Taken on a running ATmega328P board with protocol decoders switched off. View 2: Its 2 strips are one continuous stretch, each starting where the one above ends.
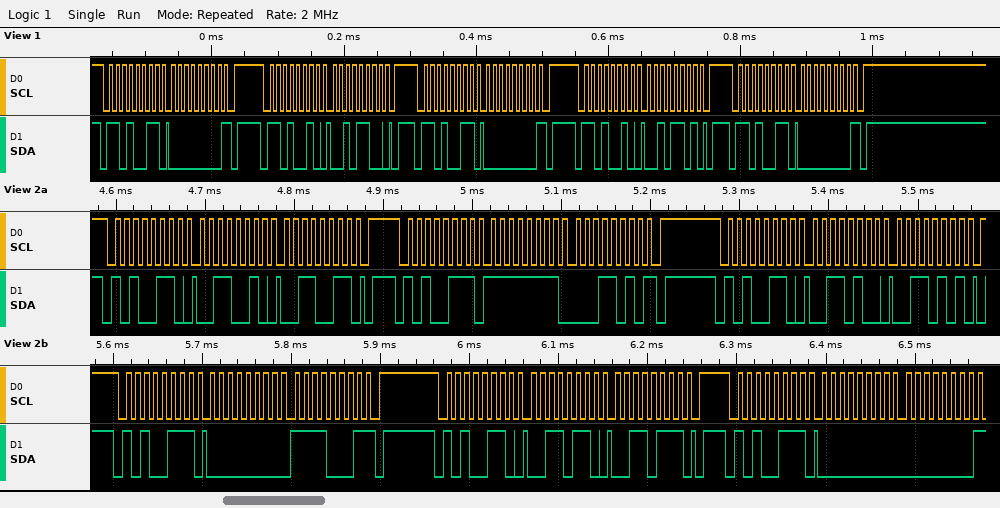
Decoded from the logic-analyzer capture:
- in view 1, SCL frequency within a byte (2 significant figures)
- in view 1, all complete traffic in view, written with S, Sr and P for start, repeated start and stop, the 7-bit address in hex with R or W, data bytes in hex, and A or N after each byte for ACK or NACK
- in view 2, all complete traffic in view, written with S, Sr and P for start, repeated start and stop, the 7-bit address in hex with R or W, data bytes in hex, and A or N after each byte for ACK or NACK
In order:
100 kHz
S 69R A 00 N P S 69W A 2C A P S 69R A 00 N P S 69W A 2D A P S 69R A 00 N P
S 53W A 32 A 33 A P S 53R A FF A 1A N P S 53W A 34 A 35 A P S 53R A 00 A F1 N P S 53W A 36 A 37 A P S 53R A 00 A 00 N
